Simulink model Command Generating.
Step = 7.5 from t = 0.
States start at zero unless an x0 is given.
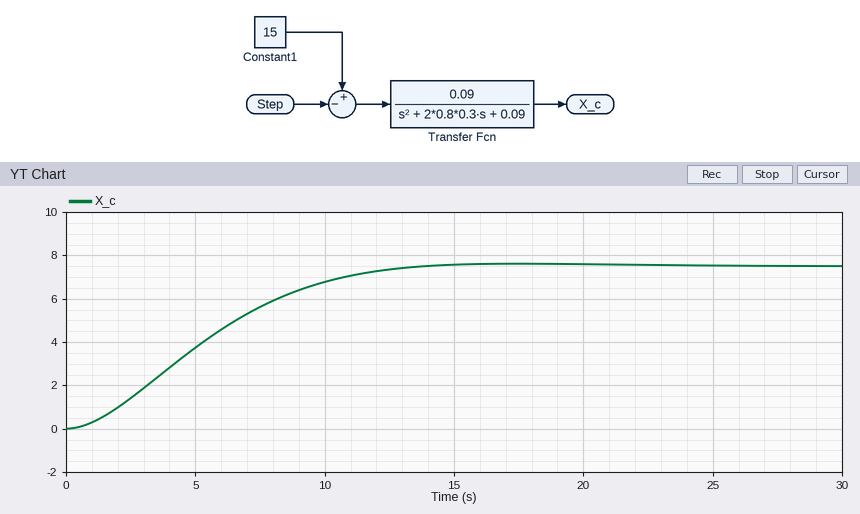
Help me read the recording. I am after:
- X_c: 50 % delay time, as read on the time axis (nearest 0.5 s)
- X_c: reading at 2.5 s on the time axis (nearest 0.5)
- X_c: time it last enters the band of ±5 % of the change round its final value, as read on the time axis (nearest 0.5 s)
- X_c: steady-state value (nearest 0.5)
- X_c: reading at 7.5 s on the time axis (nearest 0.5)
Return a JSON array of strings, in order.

["5.0 s", "1.5", "11.5 s", "7.5", "5.5"]
